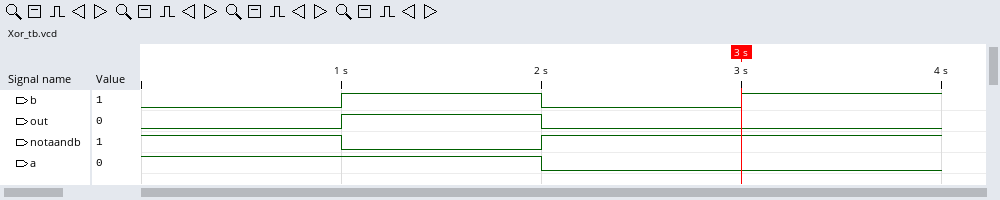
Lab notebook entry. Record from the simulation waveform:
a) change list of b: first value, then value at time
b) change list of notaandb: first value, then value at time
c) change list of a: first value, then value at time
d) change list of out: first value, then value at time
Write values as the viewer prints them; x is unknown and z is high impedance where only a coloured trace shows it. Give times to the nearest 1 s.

0, 1 at 1 s, 0 at 2 s, 1 at 3 s
1, 0 at 1 s, 1 at 2 s
1, 0 at 2 s
0, 1 at 1 s, 0 at 2 s
